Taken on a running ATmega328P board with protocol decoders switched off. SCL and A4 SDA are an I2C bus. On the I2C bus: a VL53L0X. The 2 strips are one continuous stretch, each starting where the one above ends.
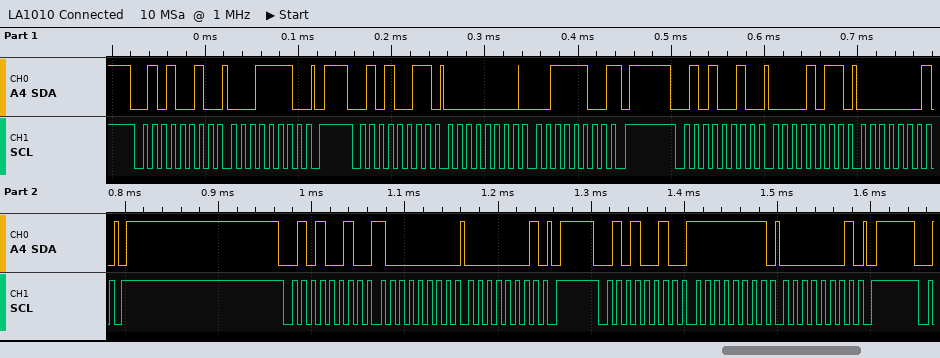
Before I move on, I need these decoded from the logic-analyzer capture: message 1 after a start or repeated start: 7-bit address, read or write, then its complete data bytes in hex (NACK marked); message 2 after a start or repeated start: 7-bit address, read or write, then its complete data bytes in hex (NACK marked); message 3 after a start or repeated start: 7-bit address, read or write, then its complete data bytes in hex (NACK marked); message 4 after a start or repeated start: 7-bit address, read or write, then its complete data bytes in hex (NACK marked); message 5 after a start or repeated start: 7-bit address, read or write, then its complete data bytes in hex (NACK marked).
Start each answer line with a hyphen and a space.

- 0x29 write: 1E
- 0x29 read: 00 3C NACK
- 0x29 write: 0B 01
- 0x29 write: 80 01
- 0x29 write: FF 01
